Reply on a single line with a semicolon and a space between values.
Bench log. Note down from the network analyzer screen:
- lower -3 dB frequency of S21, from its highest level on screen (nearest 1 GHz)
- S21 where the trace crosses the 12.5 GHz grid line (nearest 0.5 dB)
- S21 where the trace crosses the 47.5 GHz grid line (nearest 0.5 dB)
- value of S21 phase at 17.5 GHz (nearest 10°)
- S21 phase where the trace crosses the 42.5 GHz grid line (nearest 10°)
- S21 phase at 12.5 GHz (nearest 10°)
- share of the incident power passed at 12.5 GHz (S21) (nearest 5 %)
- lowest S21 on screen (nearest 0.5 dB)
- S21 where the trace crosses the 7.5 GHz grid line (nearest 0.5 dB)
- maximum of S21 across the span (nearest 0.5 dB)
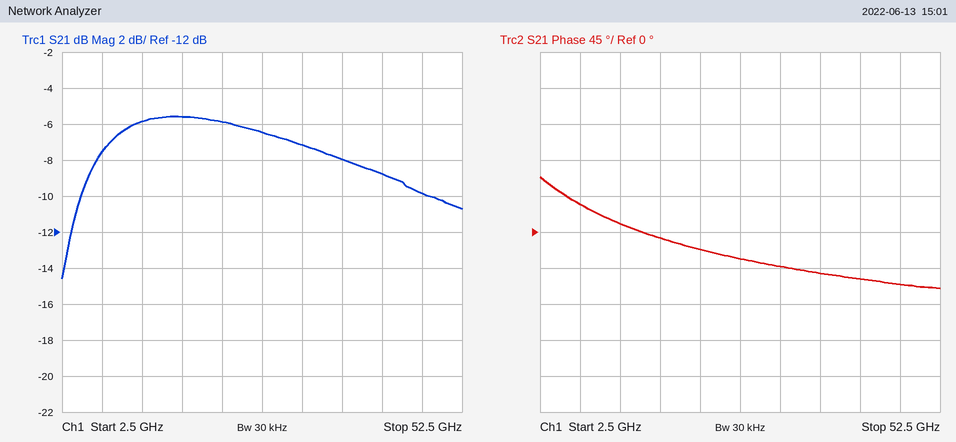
6 GHz; -6.0 dB; -10.0 dB; -10°; -60°; 10°; 25 %; -14.5 dB; -7.5 dB; -5.5 dB
